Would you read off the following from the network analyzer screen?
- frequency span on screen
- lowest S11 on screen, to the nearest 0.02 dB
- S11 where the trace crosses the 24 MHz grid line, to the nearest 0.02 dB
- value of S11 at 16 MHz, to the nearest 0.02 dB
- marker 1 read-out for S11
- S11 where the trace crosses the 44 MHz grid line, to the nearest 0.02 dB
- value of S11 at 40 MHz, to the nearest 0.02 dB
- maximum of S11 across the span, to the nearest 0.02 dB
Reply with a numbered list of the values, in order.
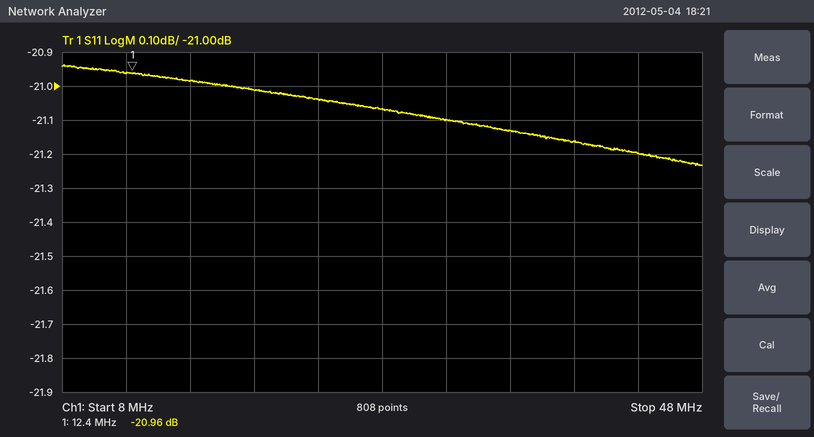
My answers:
1. 40 MHz
2. -21.24 dB
3. -21.04 dB
4. -20.98 dB
5. -20.96 dB
6. -21.20 dB
7. -21.16 dB
8. -20.94 dB
